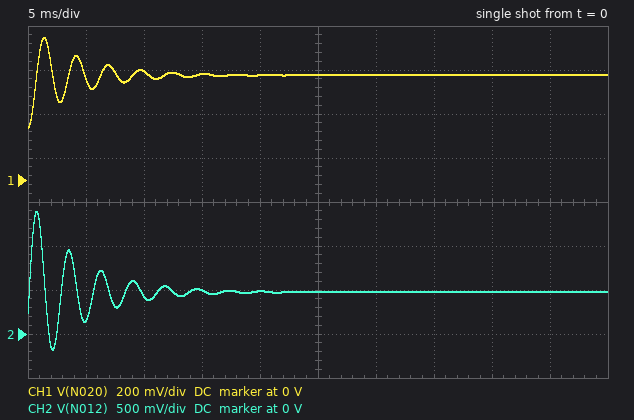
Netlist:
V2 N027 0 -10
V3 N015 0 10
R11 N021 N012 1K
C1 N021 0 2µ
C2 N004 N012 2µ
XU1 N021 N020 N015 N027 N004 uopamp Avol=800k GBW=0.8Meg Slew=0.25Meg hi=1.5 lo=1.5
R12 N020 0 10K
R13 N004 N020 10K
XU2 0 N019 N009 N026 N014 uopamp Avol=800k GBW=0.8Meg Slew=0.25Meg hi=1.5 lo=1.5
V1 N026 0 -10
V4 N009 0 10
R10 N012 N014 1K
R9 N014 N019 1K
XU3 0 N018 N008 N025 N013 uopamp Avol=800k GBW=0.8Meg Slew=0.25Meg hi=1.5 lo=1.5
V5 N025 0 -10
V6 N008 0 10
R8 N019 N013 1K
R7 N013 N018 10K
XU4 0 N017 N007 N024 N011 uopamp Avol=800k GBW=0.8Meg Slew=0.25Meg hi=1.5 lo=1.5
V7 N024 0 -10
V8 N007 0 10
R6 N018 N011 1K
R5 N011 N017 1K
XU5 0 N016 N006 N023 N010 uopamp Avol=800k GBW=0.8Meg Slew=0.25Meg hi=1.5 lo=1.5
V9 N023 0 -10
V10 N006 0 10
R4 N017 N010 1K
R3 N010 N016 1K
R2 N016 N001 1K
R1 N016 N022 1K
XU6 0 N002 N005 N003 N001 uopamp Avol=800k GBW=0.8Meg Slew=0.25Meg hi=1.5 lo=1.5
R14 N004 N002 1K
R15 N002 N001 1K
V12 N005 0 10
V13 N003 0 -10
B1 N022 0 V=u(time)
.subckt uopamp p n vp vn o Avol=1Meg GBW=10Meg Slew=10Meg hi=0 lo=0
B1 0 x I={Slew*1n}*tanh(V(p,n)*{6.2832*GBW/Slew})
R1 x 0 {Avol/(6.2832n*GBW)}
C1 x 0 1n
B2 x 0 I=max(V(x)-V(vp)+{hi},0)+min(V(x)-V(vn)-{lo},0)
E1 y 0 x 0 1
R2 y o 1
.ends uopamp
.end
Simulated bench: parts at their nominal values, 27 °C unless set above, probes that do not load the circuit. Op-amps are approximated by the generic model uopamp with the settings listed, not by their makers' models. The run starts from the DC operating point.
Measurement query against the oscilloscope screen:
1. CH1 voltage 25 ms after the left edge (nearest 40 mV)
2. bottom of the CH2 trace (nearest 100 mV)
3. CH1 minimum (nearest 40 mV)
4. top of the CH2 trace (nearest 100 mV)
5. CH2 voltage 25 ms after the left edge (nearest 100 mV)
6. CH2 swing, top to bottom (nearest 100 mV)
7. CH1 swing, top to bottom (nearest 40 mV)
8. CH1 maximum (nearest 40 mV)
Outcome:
480 mV
-200 mV
240 mV
1.4 V
500 mV
1.6 V
400 mV
640 mV
